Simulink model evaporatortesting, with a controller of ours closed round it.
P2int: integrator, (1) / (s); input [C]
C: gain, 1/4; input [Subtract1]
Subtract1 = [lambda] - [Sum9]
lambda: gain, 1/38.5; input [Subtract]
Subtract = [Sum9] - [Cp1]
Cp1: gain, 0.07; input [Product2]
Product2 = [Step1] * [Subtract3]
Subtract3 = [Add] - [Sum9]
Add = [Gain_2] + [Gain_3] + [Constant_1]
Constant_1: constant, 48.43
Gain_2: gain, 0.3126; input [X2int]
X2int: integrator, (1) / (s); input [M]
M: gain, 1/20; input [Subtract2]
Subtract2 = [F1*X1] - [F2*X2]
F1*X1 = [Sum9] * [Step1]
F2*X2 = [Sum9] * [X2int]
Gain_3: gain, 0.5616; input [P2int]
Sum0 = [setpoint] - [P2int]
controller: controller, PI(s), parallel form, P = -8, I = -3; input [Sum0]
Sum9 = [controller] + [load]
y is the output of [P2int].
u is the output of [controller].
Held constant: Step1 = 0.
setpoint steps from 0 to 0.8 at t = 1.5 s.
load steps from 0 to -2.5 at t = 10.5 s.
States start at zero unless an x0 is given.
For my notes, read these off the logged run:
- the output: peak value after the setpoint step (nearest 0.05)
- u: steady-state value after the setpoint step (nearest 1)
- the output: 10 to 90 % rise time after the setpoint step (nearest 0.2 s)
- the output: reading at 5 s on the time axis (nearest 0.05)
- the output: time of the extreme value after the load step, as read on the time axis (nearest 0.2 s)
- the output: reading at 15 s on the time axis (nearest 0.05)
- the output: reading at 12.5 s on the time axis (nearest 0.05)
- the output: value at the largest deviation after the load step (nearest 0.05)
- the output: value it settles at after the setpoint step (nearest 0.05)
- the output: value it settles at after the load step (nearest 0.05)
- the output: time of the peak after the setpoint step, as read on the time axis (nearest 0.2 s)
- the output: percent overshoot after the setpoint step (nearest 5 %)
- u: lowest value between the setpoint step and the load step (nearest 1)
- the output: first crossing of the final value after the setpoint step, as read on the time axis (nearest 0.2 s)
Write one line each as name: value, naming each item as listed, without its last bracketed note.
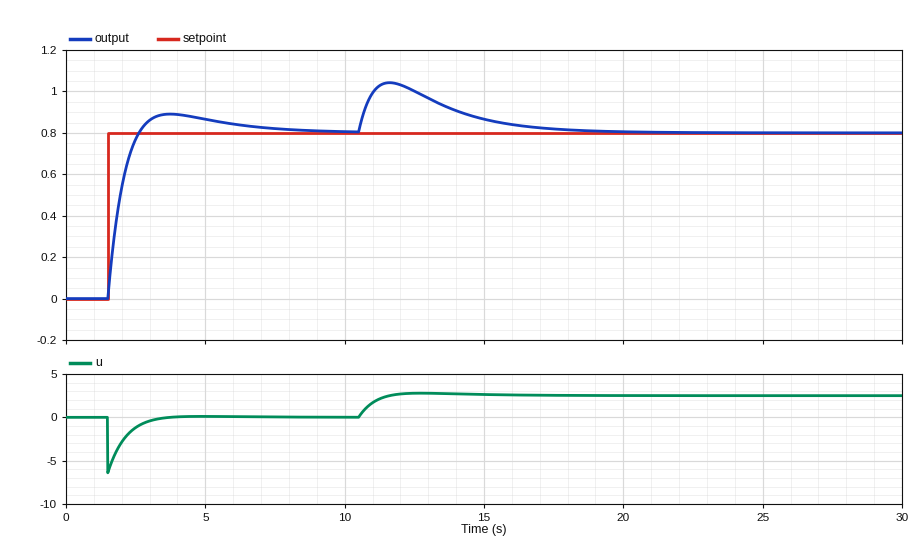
the output: peak value after the setpoint step: 0.90
u: steady-state value after the setpoint step: 0
the output: 10 to 90 % rise time after the setpoint step: 0.8 s
the output: reading at 5 s on the time axis: 0.85
the output: time of the extreme value after the load step, as read on the time axis: 11.6 s
the output: reading at 15 s on the time axis: 0.85
the output: reading at 12.5 s on the time axis: 1.00
the output: value at the largest deviation after the load step: 1.05
the output: value it settles at after the setpoint step: 0.80
the output: value it settles at after the load step: 0.80
the output: time of the peak after the setpoint step, as read on the time axis: 3.8 s
the output: percent overshoot after the setpoint step: 10 %
u: lowest value between the setpoint step and the load step: -6
the output: first crossing of the final value after the setpoint step, as read on the time axis: 2.6 s
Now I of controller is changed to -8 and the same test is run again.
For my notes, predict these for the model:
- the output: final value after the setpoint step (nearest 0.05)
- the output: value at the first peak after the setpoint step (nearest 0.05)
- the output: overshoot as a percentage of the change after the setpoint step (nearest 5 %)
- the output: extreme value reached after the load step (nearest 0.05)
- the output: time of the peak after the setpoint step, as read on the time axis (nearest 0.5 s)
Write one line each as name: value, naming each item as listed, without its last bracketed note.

the output: final value after the setpoint step: 0.80
the output: value at the first peak after the setpoint step: 0.95
the output: overshoot as a percentage of the change after the setpoint step: 20 %
the output: extreme value reached after the load step: 1.00
the output: time of the peak after the setpoint step, as read on the time axis: 3.0 s
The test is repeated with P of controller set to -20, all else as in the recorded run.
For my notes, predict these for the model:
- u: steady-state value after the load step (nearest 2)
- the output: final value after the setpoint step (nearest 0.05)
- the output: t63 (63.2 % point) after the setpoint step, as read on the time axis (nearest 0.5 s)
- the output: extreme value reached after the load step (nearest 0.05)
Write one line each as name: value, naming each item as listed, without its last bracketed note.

u: steady-state value after the load step: 2
the output: final value after the setpoint step: 0.80
the output: t63 (63.2 % point) after the setpoint step, as read on the time axis: 1.5 s
the output: extreme value reached after the load step: 0.90
